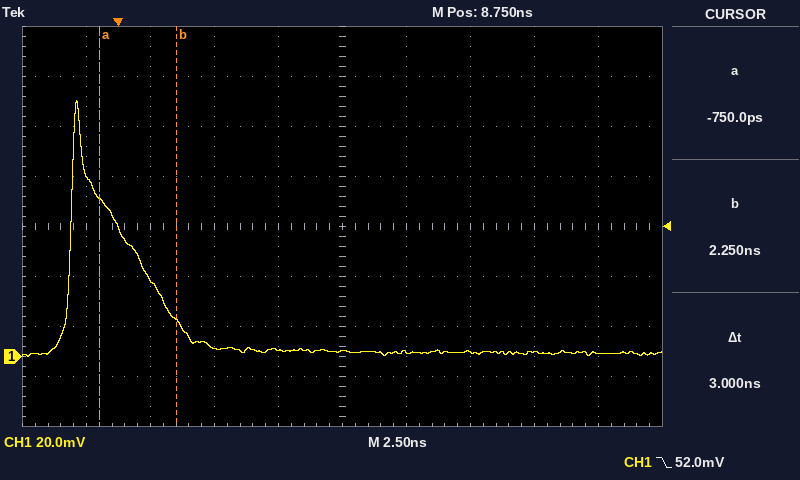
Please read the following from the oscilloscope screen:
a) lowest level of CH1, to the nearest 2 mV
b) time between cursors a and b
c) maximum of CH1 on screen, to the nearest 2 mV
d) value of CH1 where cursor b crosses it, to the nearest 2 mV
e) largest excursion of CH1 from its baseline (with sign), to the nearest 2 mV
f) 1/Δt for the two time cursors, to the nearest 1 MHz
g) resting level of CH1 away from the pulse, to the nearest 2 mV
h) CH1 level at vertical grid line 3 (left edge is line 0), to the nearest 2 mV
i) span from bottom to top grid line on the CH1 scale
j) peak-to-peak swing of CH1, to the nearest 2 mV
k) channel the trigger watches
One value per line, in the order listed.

0 mV
3 ns
102 mV
14 mV
+100 mV
333 MHz
2 mV
4 mV
160 mV
102 mV
CH1
